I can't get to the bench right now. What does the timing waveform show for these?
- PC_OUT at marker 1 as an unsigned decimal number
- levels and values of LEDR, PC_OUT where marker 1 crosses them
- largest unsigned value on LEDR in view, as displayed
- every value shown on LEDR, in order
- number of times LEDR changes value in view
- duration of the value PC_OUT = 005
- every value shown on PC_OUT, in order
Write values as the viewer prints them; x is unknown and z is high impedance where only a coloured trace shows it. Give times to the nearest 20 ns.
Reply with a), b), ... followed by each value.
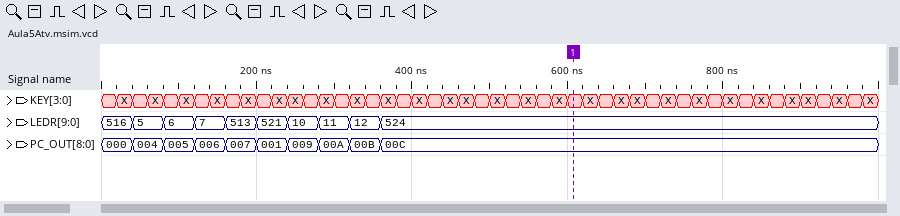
a) 12
b) LEDR=524, PC_OUT=00C
c) 524
d) 516, 5, 6, 7, 513, 521, 10, 11, 12, 524
e) 9
f) 40 ns
g) 000, 004, 005, 006, 007, 001, 009, 00A, 00B, 00C
